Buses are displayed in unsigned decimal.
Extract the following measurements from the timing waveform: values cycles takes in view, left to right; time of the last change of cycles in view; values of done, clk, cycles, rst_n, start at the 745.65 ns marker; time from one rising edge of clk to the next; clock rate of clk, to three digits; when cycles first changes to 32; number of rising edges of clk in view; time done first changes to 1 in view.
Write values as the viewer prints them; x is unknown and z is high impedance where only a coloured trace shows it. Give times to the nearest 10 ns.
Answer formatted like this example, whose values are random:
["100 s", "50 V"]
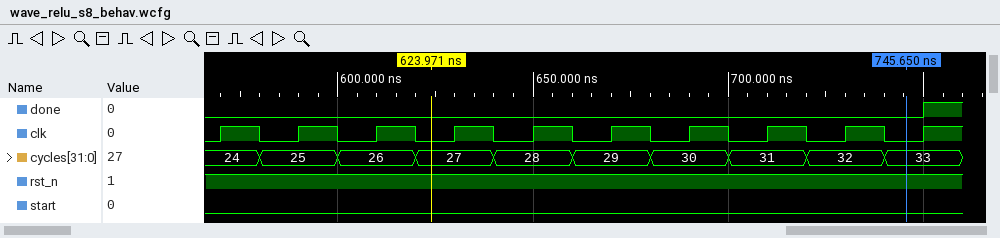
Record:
["24, 25, 26, 27, 28, 29, 30, 31, 32, 33", "740 ns", "done=0, clk=0, cycles=33, rst_n=1, start=0", "20 ns", "50.0 MHz", "720 ns", "10", "750 ns"]
